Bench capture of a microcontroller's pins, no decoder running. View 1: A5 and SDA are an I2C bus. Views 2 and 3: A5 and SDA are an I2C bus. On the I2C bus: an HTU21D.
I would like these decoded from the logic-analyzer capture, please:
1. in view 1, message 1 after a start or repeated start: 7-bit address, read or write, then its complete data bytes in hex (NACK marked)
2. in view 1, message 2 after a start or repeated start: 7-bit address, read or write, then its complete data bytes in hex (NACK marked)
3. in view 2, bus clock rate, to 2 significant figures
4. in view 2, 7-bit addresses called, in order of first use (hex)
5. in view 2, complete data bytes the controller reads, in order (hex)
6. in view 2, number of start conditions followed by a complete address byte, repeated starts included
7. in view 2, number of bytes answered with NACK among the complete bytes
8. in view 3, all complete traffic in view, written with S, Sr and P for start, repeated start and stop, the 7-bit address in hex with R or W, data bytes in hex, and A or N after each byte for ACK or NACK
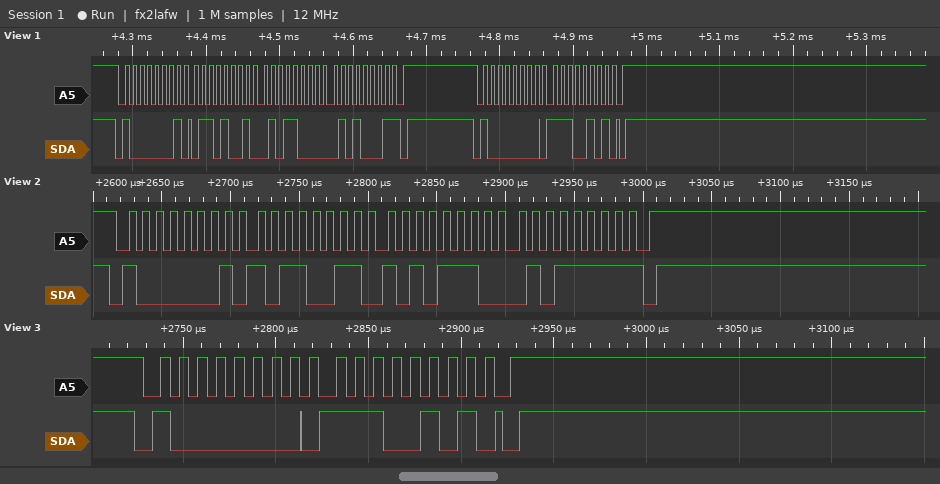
0x40 read: 69 58 51 NACK
0x40 write: E5
100 kHz
0x40
B3 AE 5F
1
1
S 40W A E5 A P
